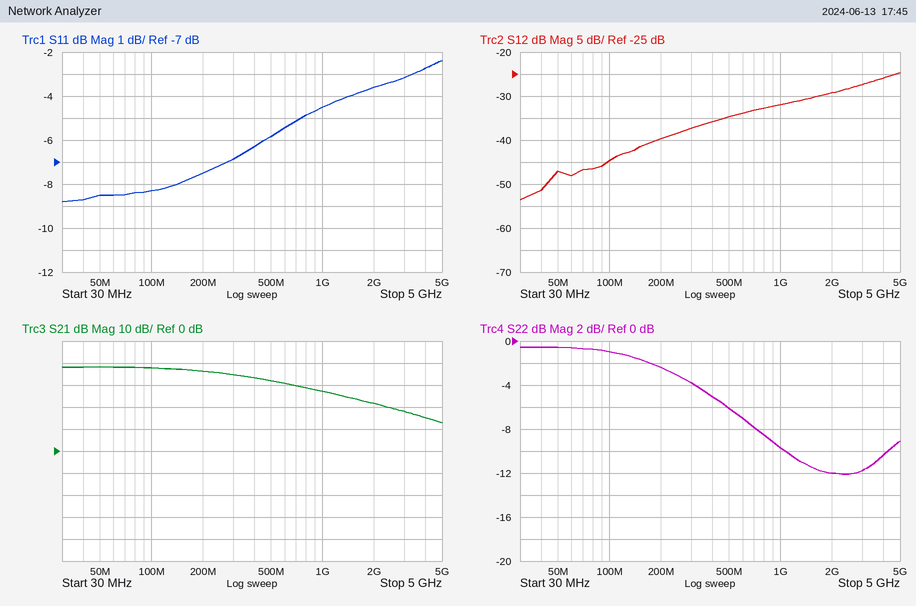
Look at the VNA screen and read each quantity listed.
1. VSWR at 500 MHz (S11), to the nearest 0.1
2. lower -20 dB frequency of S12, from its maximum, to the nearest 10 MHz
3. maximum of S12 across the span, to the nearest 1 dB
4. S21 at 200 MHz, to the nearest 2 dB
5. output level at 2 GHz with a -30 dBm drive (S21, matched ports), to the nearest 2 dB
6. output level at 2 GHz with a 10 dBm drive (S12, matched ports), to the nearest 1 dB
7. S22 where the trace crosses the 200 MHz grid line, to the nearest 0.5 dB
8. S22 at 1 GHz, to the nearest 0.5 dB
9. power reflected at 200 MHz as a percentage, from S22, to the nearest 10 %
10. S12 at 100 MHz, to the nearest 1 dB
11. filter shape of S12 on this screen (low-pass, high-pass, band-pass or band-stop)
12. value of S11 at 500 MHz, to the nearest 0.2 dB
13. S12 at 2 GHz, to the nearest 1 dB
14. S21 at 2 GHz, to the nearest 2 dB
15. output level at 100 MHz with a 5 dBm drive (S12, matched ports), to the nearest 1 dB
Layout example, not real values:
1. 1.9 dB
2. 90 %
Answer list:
1. 3.1
2. 100 MHz
3. -25 dB
4. 36 dB
5. -8 dBm
6. -19 dBm
7. -2.5 dB
8. -9.5 dB
9. 60 %
10. -45 dB
11. high-pass
12. -5.8 dB
13. -29 dB
14. 22 dB
15. -40 dBm
